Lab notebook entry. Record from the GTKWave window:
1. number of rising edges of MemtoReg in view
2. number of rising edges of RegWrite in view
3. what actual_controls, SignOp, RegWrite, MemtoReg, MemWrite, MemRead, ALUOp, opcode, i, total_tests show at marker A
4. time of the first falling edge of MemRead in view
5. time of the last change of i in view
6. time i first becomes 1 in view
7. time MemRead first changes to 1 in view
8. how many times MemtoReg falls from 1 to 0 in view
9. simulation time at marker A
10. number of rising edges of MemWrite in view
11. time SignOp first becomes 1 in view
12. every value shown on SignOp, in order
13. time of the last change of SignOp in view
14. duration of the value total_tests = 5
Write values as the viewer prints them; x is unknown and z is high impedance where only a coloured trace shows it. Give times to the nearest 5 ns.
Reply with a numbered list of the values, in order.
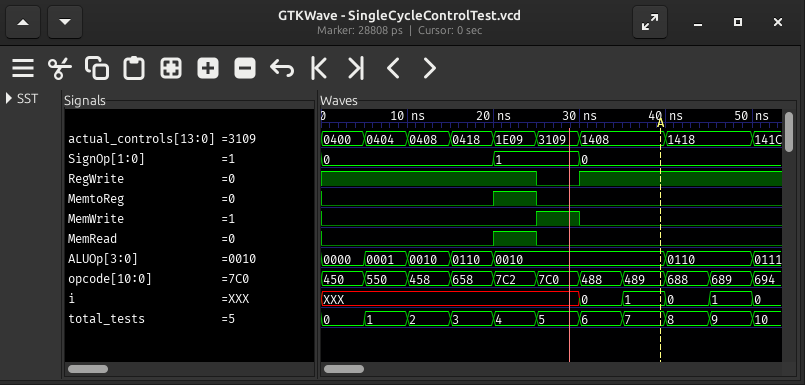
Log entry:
1. 1
2. 1
3. actual_controls=1408, SignOp=0, RegWrite=1, MemtoReg=0, MemWrite=0, MemRead=0, ALUOp=0010, opcode=489, i=1, total_tests=7
4. 25 ns
5. 50 ns
6. 35 ns
7. 20 ns
8. 1
9. 40 ns
10. 1
11. 20 ns
12. 0, 1, 0
13. 30 ns
14. 5 ns
